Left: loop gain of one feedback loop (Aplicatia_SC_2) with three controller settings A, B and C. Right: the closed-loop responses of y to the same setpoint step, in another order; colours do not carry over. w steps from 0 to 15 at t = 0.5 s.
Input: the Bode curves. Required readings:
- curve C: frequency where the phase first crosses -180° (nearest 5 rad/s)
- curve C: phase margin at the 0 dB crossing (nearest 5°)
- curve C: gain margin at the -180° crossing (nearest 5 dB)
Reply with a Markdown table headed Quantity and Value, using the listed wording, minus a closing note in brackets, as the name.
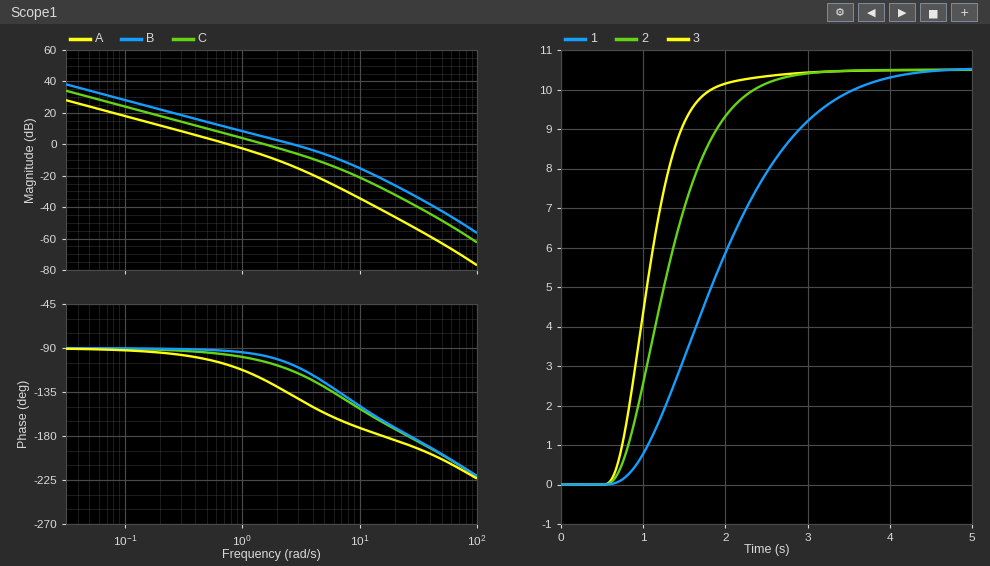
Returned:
| Quantity | Value |
|---|---|
| curve C: frequency where the phase first crosses -180° | 25 rad/s |
| curve C: phase margin at the 0 dB crossing | 75° |
| curve C: gain margin at the -180° crossing | 35 dB |
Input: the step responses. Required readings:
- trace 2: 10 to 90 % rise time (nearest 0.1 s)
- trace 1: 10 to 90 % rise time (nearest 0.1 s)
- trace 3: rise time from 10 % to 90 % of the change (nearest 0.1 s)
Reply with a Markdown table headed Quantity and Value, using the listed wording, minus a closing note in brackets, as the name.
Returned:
| Quantity | Value |
|---|---|
| trace 2: 10 to 90 % rise time | 1.2 s |
| trace 1: 10 to 90 % rise time | 2.1 s |
| trace 3: rise time from 10 % to 90 % of the change | 0.8 s |
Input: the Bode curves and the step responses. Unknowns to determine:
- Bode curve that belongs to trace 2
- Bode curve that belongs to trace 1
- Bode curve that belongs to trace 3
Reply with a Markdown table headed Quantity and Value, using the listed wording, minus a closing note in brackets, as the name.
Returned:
| Quantity | Value |
|---|---|
| Bode curve that belongs to trace 2 | C |
| Bode curve that belongs to trace 1 | A |
| Bode curve that belongs to trace 3 | B |
